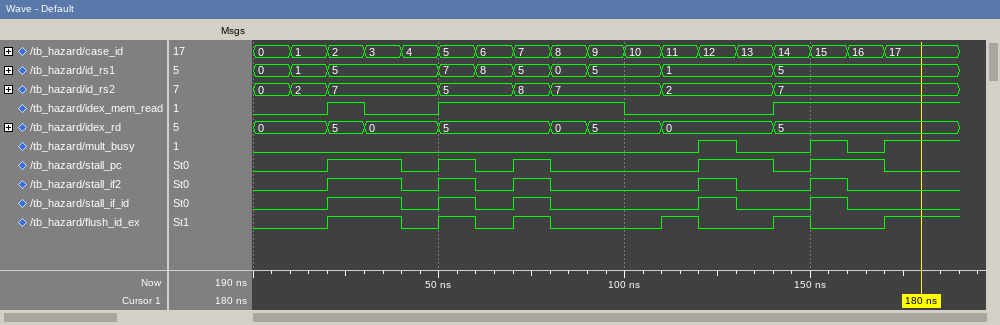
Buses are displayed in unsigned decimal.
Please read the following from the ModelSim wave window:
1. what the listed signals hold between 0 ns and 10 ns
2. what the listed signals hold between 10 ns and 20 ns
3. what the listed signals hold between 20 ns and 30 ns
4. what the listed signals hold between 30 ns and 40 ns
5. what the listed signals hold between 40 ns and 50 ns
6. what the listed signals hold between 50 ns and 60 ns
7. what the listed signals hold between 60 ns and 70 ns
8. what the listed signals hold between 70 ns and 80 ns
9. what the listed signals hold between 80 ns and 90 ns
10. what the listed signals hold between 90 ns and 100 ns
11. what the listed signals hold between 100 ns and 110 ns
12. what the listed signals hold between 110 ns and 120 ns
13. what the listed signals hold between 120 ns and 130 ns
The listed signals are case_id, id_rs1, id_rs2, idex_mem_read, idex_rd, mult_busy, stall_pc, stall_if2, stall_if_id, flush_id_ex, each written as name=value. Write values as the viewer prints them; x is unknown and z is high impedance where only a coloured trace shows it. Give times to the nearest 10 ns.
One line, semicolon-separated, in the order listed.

case_id=0, id_rs1=0, id_rs2=0, idex_mem_read=0, idex_rd=0, mult_busy=0, stall_pc=0, stall_if2=0, stall_if_id=0, flush_id_ex=0; case_id=1, id_rs1=1, id_rs2=2, idex_mem_read=0, idex_rd=0, mult_busy=0, stall_pc=0, stall_if2=0, stall_if_id=0, flush_id_ex=0; case_id=2, id_rs1=5, id_rs2=7, idex_mem_read=1, idex_rd=5, mult_busy=0, stall_pc=1, stall_if2=1, stall_if_id=1, flush_id_ex=1; case_id=3, id_rs1=5, id_rs2=7, idex_mem_read=0, idex_rd=0, mult_busy=0, stall_pc=1, stall_if2=1, stall_if_id=1, flush_id_ex=1; case_id=4, id_rs1=5, id_rs2=7, idex_mem_read=0, idex_rd=0, mult_busy=0, stall_pc=0, stall_if2=0, stall_if_id=0, flush_id_ex=0; case_id=5, id_rs1=7, id_rs2=5, idex_mem_read=1, idex_rd=5, mult_busy=0, stall_pc=1, stall_if2=1, stall_if_id=1, flush_id_ex=1; case_id=6, id_rs1=8, id_rs2=5, idex_mem_read=1, idex_rd=5, mult_busy=0, stall_pc=0, stall_if2=0, stall_if_id=0, flush_id_ex=0; case_id=7, id_rs1=5, id_rs2=8, idex_mem_read=1, idex_rd=5, mult_busy=0, stall_pc=1, stall_if2=1, stall_if_id=1, flush_id_ex=1; case_id=8, id_rs1=0, id_rs2=7, idex_mem_read=1, idex_rd=0, mult_busy=0, stall_pc=0, stall_if2=0, stall_if_id=0, flush_id_ex=0; case_id=9, id_rs1=5, id_rs2=7, idex_mem_read=1, idex_rd=5, mult_busy=0, stall_pc=0, stall_if2=0, stall_if_id=0, flush_id_ex=0; case_id=10, id_rs1=5, id_rs2=7, idex_mem_read=0, idex_rd=5, mult_busy=0, stall_pc=0, stall_if2=0, stall_if_id=0, flush_id_ex=0; case_id=11, id_rs1=1, id_rs2=2, idex_mem_read=0, idex_rd=0, mult_busy=0, stall_pc=0, stall_if2=0, stall_if_id=0, flush_id_ex=1; case_id=12, id_rs1=1, id_rs2=2, idex_mem_read=0, idex_rd=0, mult_busy=1, stall_pc=1, stall_if2=1, stall_if_id=1, flush_id_ex=0
